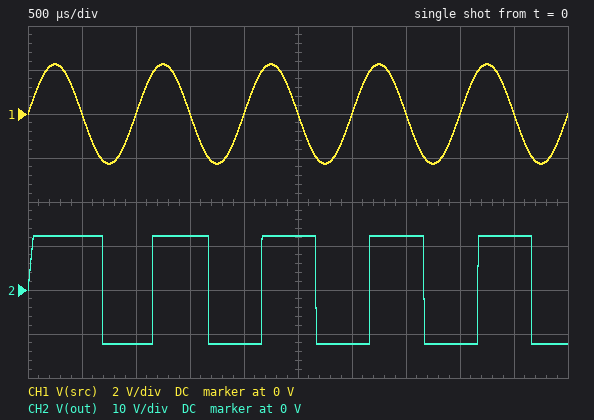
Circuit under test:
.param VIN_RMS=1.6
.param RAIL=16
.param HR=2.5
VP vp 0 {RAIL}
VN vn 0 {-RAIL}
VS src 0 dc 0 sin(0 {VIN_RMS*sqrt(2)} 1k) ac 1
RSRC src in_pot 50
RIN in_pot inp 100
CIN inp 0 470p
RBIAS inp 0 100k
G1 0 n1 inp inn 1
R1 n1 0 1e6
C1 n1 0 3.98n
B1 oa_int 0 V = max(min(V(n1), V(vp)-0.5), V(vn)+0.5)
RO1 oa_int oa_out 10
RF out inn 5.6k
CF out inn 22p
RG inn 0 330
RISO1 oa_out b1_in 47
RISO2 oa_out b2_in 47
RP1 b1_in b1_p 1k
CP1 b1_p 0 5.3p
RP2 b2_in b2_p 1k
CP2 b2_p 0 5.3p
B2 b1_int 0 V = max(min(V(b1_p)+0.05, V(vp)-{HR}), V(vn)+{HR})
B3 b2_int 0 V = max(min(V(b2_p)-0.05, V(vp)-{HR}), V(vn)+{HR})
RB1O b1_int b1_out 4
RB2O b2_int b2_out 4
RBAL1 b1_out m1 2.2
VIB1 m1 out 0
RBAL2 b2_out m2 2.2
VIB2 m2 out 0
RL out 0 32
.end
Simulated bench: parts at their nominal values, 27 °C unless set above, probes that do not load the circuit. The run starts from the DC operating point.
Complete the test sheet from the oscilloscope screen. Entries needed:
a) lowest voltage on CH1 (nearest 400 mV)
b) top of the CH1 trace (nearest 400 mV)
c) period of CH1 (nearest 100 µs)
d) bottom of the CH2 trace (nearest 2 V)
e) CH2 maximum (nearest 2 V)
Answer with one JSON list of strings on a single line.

["-2.4 V", "2.4 V", "1.0 ms", "-12 V", "12 V"]
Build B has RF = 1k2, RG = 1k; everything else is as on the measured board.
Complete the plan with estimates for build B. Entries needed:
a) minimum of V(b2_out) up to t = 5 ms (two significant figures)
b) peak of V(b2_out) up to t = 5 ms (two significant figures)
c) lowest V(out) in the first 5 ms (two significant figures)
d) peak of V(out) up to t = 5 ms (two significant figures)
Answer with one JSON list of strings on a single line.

["-5.2 V", "5.1 V", "-5.0 V", "5.0 V"]
